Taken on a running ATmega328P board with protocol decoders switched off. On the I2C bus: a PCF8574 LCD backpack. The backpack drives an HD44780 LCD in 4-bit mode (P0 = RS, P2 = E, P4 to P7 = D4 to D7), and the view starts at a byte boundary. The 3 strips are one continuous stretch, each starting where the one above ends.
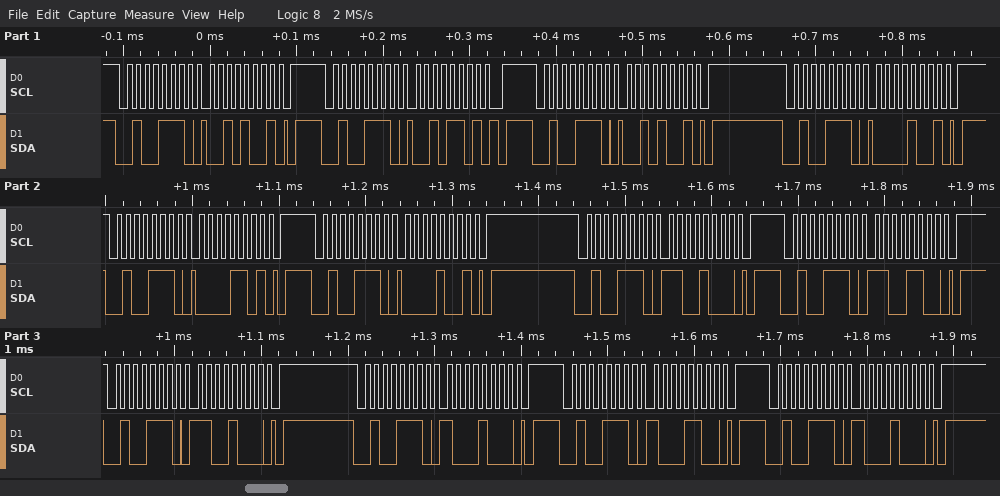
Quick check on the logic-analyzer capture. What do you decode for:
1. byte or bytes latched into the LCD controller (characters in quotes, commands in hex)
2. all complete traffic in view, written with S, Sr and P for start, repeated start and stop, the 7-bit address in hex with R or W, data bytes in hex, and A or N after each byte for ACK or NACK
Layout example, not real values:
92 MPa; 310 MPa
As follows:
' ' 0xC8; S 27W A 29 A P S 27W A 2D A P S 27W A 29 A P S 27W A 09 A P S 27W A 0D A P S 27W A 09 A P S 27W A C8 A P S 27W A CC A P S 27W A C8 A P S 27W A 88 A P S 27W A 8C A P S 27W A 88 A P
